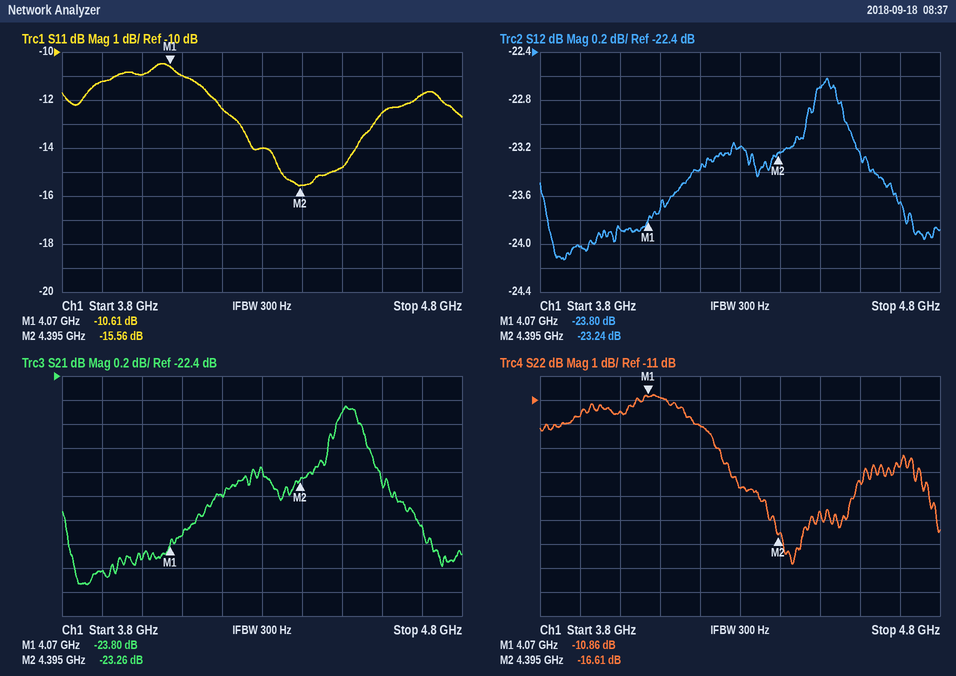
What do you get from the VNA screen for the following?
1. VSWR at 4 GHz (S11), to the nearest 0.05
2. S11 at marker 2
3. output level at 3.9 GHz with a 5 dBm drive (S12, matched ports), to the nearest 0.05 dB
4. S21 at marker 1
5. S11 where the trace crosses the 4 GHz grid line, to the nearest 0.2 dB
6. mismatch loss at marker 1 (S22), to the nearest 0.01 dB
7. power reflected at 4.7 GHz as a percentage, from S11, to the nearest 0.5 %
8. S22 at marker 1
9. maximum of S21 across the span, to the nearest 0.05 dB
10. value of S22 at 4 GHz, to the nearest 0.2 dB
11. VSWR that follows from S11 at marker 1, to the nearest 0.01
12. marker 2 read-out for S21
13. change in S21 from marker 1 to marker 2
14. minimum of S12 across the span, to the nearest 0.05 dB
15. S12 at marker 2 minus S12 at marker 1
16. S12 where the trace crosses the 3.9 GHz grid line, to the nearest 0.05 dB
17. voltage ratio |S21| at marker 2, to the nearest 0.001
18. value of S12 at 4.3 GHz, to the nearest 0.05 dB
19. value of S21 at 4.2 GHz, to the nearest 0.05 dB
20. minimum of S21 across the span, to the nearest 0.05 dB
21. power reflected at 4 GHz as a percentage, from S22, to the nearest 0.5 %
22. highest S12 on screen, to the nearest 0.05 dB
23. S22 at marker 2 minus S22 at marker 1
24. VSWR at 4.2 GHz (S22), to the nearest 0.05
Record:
1.80
-15.56 dB
-19.00 dBm
-23.80 dB
-11.0 dB
0.37 dB
6.5 %
-10.86 dB
-22.65 dB
-11.4 dB
1.84
-23.26 dB
0.54 dB
-24.15 dB
0.56 dB
-24.00 dB
0.069
-23.20 dB
-23.40 dB
-24.15 dB
7.0 %
-22.60 dB
-5.75 dB
1.65
